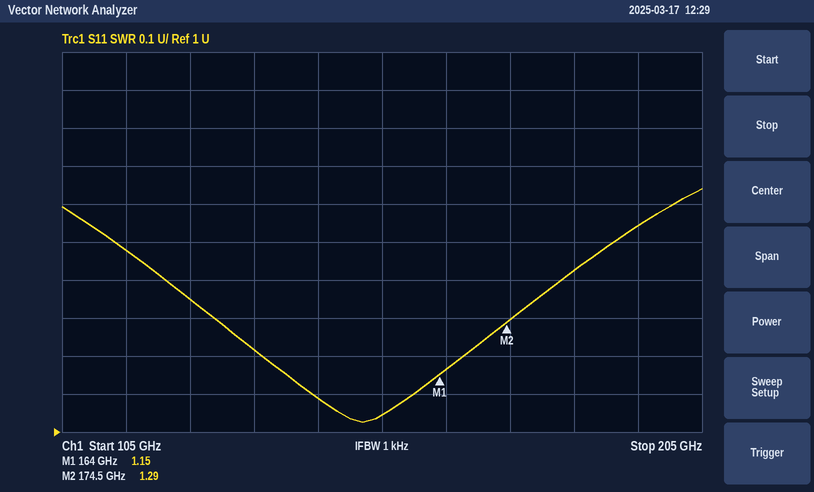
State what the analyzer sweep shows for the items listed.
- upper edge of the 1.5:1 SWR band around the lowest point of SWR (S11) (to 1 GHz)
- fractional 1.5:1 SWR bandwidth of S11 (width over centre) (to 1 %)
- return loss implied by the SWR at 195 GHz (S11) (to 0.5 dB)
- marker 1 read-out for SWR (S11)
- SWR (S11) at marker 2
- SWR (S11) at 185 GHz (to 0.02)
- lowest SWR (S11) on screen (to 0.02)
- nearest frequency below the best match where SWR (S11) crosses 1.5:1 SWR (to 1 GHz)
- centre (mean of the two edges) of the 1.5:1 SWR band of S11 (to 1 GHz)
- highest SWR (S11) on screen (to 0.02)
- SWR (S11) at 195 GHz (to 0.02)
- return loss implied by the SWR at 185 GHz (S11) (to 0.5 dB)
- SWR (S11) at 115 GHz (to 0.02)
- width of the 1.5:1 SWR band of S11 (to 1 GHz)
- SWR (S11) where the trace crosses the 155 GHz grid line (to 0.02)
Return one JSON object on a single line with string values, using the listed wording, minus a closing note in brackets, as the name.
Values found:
{"upper edge of the 1.5:1 SWR band around the lowest point of SWR (S11)": "191 GHz", "fractional 1.5:1 SWR bandwidth of S11 (width over centre)": "51 %", "return loss implied by the SWR at 195 GHz (S11)": "13.5 dB", "marker 1 read-out for SWR": "1.15", "SWR (S11) at marker 2": "1.29", "SWR (S11) at 185 GHz": "1.42", "lowest SWR (S11) on screen": "1.02", "nearest frequency below the best match where SWR (S11) crosses 1.5:1 SWR": "113 GHz", "centre (mean of the two edges) of the 1.5:1 SWR band of S11": "152 GHz", "highest SWR (S11) on screen": "1.64", "SWR (S11) at 195 GHz": "1.54", "return loss implied by the SWR at 185 GHz (S11)": "15.0 dB", "SWR (S11) at 115 GHz": "1.48", "width of the 1.5:1 SWR band of S11": "78 GHz", "SWR (S11) where the trace crosses the 155 GHz grid line": "1.04"}
